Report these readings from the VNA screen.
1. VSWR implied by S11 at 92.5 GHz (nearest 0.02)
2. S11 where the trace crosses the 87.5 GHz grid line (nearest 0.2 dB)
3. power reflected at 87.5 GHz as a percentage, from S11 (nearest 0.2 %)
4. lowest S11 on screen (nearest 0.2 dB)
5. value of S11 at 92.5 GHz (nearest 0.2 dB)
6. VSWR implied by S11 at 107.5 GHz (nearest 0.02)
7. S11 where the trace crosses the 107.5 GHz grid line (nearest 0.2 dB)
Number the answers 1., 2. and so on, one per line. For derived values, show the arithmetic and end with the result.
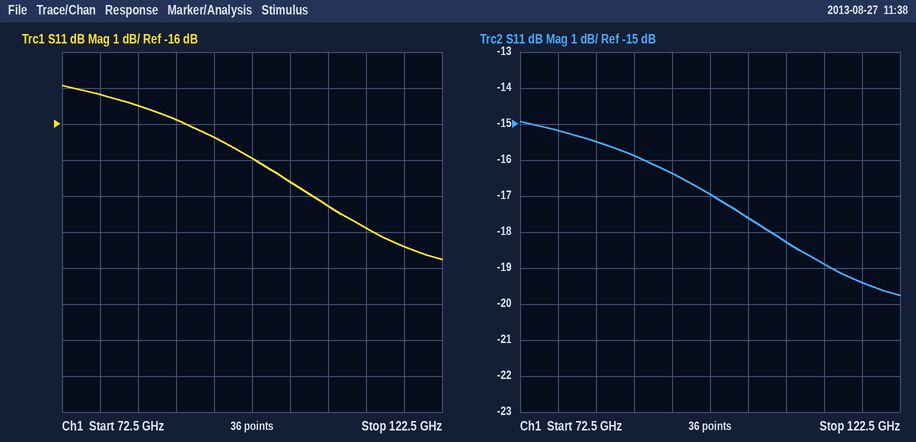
1. |Γ| = 10^(-16.4/20) = 0.1514; VSWR = (1 + 0.1514)/(1 − 0.1514) ≈ 1.36
2. -15.8 dB
3. 10^(-15.8/10) ≈ 2.6 %
4. -19.8 dB
5. -16.4 dB
6. |Γ| = 10^(-18.2/20) = 0.1230; VSWR = (1 + 0.1230)/(1 − 0.1230) ≈ 1.28
7. -18.2 dB
